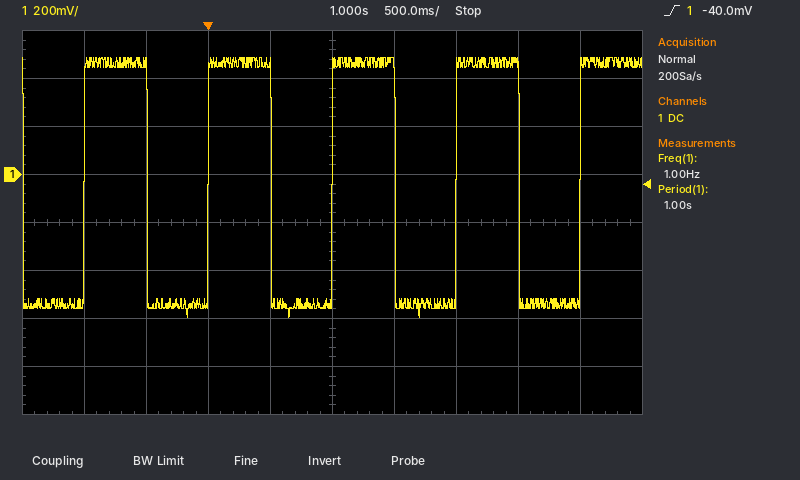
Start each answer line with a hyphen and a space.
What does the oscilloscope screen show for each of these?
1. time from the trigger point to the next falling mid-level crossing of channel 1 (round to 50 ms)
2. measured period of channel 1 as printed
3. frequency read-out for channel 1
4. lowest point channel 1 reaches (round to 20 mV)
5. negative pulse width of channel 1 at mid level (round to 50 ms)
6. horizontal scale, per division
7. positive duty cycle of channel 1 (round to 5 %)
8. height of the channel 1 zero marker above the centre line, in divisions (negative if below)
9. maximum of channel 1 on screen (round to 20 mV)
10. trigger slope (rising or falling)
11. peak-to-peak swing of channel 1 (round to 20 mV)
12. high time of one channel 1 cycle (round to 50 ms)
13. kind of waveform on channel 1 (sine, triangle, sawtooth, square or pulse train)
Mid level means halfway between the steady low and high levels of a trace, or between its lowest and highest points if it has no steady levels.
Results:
- 500 ms
- 1.00 s
- 1.00 Hz
- -600 mV
- 500 ms
- 500 ms
- 50 %
- +1.0 div
- 480 mV
- rising
- 1.08 V
- 500 ms
- square
